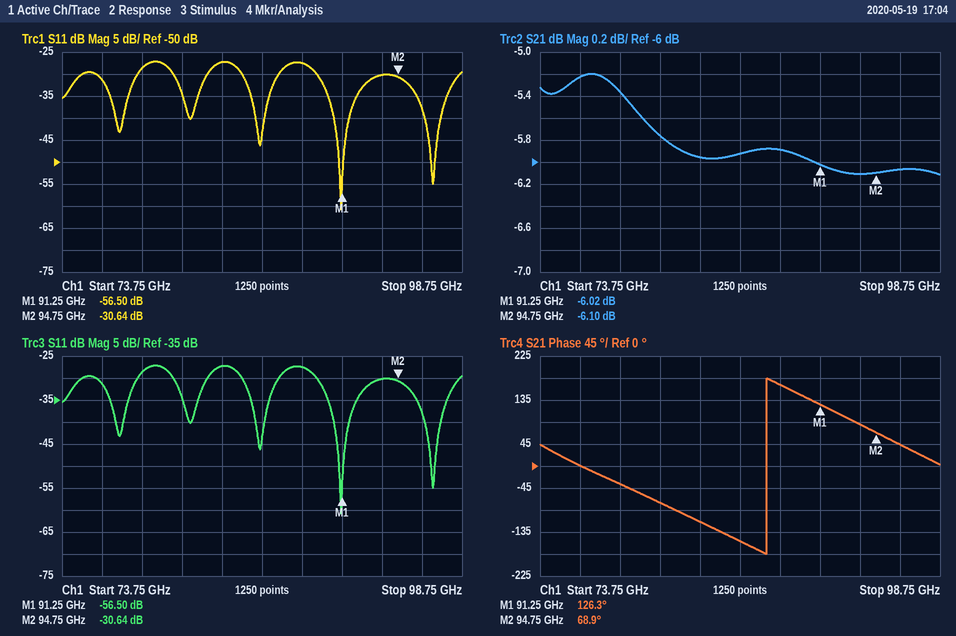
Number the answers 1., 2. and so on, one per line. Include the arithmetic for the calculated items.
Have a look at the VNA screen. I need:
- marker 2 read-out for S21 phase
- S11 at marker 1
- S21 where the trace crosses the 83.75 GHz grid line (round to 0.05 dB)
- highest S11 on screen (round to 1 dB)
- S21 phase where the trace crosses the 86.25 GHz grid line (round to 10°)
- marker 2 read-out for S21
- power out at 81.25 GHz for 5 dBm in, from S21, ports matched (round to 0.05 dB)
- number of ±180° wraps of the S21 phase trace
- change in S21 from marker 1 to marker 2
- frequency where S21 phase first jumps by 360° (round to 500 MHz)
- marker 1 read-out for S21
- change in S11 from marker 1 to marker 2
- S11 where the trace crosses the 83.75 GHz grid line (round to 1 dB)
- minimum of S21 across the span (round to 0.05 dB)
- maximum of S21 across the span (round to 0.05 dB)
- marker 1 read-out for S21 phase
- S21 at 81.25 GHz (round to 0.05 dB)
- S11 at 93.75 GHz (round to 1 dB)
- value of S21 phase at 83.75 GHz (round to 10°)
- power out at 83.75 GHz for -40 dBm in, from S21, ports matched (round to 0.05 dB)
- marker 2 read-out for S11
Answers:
1. 68.9°
2. -56.50 dB
3. -5.95 dB
4. -27 dB
5. -150°
6. -6.10 dB
7. 5 dBm + (-5.75 dB) = -0.75 dBm
8. 1
9. -6.1 − (-6.02) = -0.08 dB
10. 88.0 GHz
11. -6.02 dB
12. -30.64 − (-56.5) = 25.86 dB
13. -27 dB
14. -6.10 dB
15. -5.20 dB
16. 126.3°
17. -5.75 dB
18. -30 dB
19. -110°
20. -40 dBm + (-5.95 dB) = -45.95 dBm
21. -30.64 dB
